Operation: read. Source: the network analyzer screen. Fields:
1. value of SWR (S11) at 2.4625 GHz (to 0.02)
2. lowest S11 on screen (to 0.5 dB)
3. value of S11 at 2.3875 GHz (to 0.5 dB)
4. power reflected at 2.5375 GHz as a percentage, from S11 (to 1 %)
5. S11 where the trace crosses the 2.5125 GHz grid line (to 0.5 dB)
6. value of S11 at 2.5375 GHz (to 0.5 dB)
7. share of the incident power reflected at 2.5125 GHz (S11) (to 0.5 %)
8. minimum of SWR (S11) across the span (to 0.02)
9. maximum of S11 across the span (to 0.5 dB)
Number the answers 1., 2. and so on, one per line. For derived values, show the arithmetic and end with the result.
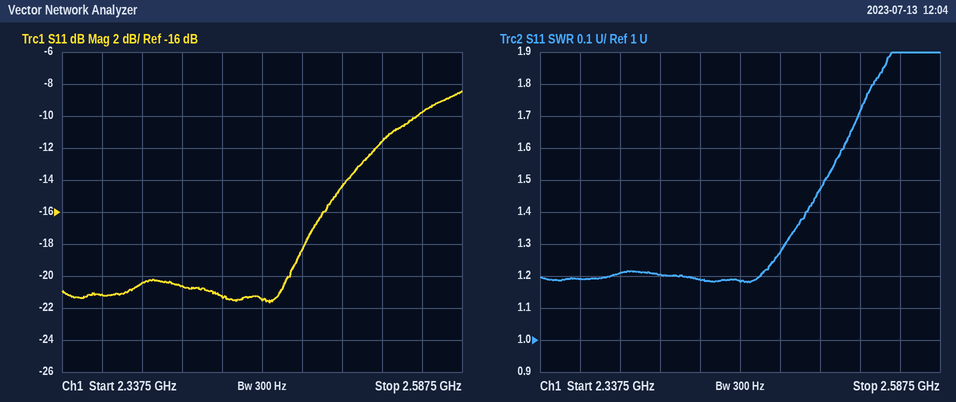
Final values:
1. 1.18
2. -21.5 dB
3. -20.5 dB
4. 10^(-11.5/10) ≈ 7 %
5. -14.5 dB
6. -11.5 dB
7. 10^(-14.5/10) ≈ 3.5 %
8. 1.18
9. -8.5 dB
